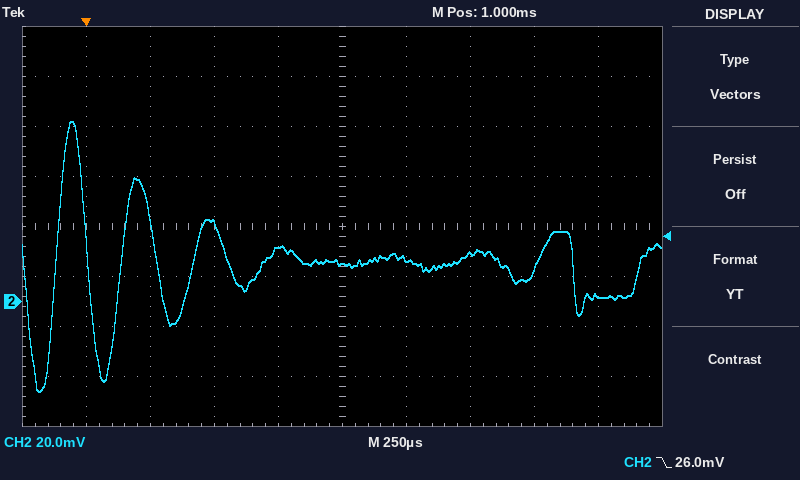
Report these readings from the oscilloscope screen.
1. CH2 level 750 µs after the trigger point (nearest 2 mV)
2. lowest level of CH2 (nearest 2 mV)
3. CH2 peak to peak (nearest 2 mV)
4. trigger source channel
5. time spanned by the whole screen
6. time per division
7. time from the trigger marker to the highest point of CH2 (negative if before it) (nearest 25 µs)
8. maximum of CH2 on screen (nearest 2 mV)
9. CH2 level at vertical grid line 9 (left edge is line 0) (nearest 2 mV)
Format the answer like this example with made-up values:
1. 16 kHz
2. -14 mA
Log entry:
1. 22 mV
2. -36 mV
3. 108 mV
4. CH2
5. 2.5 ms
6. 250 µs
7. -50 µs
8. 72 mV
9. 2 mV
